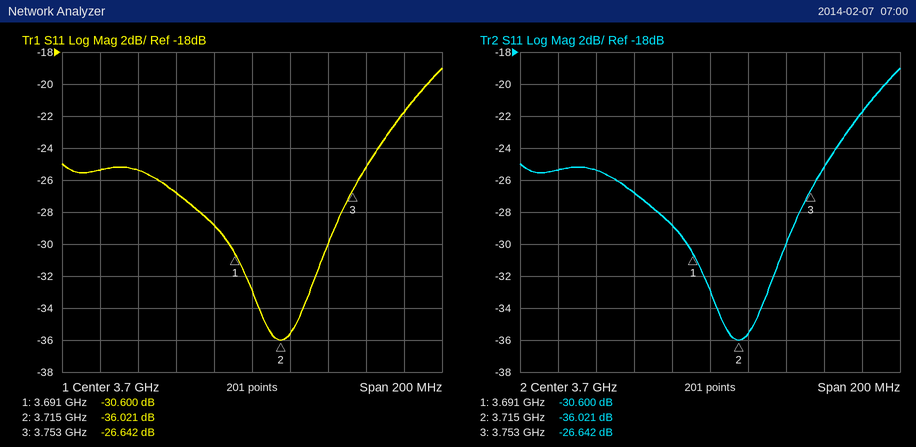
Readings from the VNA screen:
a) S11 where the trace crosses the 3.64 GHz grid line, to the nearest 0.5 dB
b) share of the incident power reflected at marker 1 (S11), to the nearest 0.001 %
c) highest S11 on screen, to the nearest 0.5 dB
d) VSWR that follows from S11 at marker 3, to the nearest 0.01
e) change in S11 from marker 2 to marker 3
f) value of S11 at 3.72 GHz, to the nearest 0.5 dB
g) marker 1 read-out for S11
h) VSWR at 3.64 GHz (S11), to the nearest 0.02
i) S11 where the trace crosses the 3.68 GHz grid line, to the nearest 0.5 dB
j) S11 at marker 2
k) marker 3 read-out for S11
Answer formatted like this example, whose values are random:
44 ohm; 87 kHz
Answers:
-25.5 dB; 0.087 %; -19.0 dB; 1.10; 9.379 dB; -35.5 dB; -30.600 dB; 1.12; -29.0 dB; -36.021 dB; -26.642 dB
